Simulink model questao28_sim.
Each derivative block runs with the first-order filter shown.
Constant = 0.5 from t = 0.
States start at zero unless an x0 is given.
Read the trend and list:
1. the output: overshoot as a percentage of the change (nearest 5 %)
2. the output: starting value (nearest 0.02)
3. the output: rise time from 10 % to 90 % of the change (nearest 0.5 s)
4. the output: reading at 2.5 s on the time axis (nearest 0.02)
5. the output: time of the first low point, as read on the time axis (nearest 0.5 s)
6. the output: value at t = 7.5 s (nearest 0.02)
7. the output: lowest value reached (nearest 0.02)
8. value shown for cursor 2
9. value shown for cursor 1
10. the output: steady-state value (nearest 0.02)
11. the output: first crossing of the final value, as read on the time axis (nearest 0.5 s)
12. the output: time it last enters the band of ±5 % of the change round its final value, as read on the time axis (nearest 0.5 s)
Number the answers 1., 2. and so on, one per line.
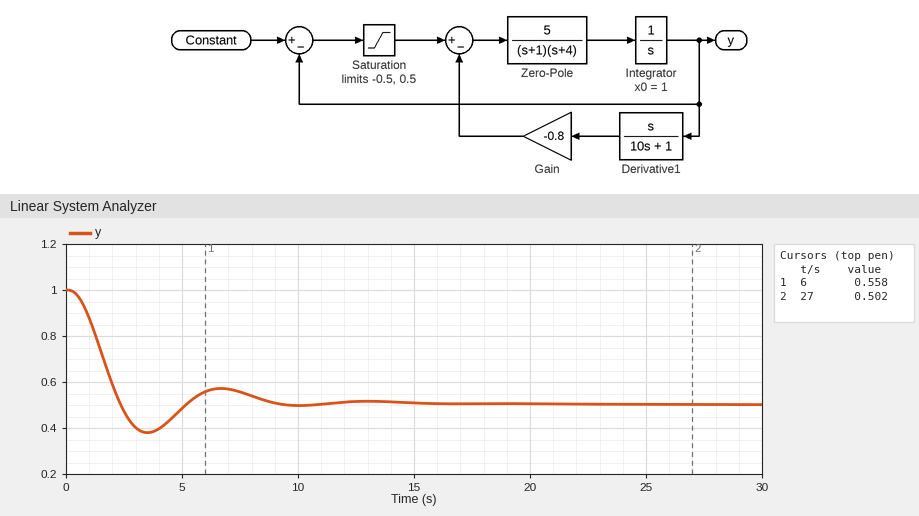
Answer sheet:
1. 25 %
2. 1.00
3. 1.5 s
4. 0.48
5. 3.5 s
6. 0.56
7. 0.38
8. 0.502
9. 0.558
10. 0.50
11. 2.5 s
12. 8.5 s
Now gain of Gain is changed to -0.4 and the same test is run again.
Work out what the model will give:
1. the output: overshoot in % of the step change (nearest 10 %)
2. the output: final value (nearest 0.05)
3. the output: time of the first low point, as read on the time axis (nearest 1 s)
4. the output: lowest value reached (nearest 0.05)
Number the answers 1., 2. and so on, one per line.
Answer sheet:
1. 30 %
2. 0.50
3. 3 s
4. 0.35
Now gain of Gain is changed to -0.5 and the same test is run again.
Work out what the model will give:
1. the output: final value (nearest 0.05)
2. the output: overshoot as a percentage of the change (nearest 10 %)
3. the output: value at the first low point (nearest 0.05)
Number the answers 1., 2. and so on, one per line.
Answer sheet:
1. 0.50
2. 30 %
3. 0.35
